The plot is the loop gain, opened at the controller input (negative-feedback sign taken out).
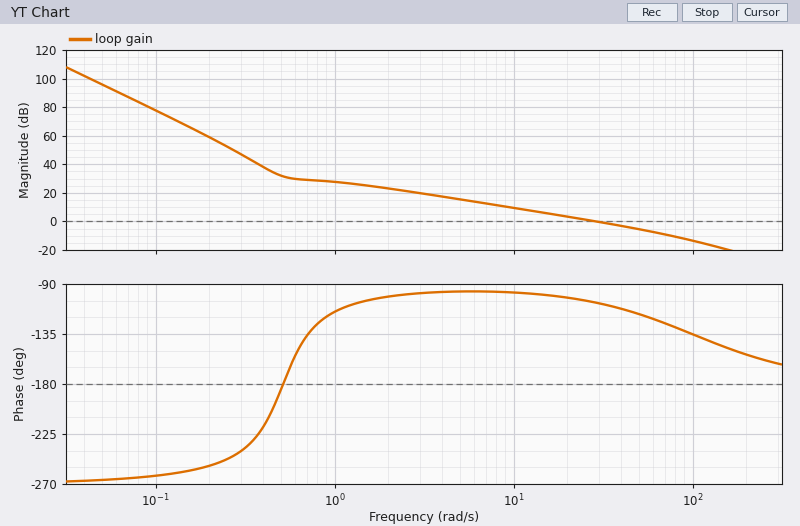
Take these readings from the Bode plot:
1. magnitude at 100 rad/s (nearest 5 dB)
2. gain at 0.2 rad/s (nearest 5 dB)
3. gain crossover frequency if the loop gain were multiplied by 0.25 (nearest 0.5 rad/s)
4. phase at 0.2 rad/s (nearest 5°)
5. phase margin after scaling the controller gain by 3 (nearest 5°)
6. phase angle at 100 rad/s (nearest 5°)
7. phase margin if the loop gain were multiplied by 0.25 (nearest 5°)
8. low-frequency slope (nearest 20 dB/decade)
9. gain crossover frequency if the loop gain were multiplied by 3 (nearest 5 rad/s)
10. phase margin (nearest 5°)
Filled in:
-15 dB
60 dB
7.5 rad/s
-255°
55°
-135°
85°
-60 dB/decade
75 rad/s
75°
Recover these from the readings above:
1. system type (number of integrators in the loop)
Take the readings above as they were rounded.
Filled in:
3
